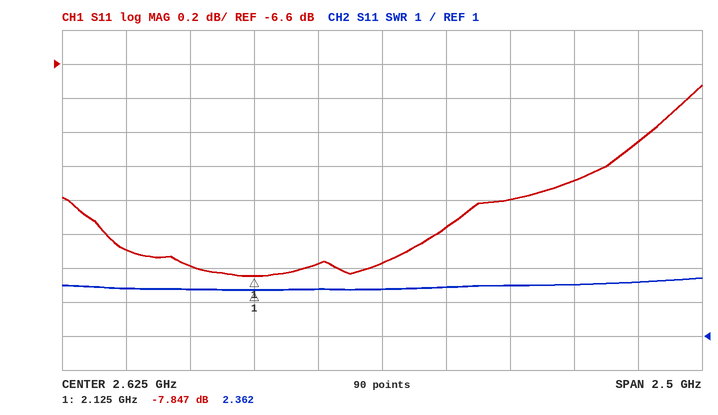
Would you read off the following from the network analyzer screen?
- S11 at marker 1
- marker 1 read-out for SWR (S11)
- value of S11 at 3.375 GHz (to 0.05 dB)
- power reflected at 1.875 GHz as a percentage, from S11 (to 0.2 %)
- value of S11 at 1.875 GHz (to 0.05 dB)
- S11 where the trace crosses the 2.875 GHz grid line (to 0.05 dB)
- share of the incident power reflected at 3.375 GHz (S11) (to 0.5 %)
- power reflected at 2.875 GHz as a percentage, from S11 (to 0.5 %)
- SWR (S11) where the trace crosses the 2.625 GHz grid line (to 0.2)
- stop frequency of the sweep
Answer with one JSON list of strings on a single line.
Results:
["-7.847 dB", "2.362", "-7.30 dB", "16.6 %", "-7.80 dB", "-7.55 dB", "18.5 %", "17.5 %", "2.4", "3.875 GHz"]
